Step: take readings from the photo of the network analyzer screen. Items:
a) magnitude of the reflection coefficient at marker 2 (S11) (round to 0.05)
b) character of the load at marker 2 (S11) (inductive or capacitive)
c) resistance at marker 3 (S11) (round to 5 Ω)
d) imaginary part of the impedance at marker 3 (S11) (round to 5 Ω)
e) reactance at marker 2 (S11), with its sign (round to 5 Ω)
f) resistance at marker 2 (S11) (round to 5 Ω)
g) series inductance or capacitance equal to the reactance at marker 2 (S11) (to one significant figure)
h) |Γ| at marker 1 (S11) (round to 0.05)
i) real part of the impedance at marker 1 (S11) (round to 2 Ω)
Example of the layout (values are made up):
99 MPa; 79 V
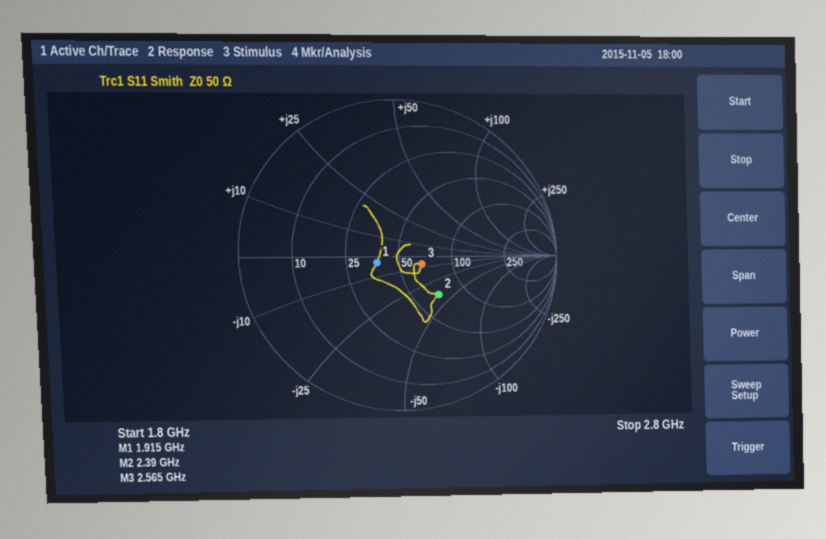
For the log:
0.35; capacitive; 65 Ω; -5 Ω; -40 Ω; 70 Ω; 2 pF; 0.15; 38 Ω
